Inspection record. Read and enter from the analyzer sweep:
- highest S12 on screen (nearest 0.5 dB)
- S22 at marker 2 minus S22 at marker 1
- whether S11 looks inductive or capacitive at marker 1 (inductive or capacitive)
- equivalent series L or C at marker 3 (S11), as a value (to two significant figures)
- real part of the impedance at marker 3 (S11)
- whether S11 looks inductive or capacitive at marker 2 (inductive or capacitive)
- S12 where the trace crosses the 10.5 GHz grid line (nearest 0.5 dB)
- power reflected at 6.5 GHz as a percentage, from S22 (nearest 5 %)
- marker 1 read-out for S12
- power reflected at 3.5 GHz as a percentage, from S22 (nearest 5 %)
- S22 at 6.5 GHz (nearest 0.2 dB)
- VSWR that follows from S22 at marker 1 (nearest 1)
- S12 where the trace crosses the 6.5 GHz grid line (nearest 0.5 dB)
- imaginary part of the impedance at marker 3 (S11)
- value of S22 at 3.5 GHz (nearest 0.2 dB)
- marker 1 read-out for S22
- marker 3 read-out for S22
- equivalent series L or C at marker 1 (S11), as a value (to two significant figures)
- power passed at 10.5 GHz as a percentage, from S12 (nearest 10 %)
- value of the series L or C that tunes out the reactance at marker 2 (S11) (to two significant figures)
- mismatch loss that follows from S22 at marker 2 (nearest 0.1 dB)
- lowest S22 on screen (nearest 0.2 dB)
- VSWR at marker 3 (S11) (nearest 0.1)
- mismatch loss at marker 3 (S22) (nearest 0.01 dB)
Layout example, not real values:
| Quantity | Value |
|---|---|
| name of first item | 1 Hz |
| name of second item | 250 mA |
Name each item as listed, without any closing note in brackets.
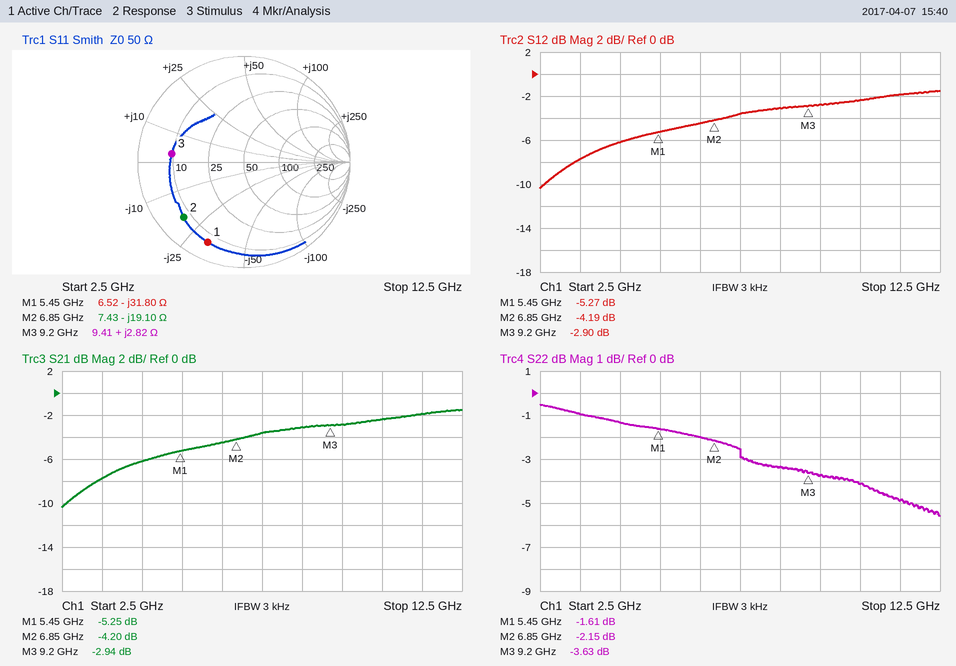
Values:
| Quantity | Value |
|---|---|
| highest S12 on screen | -1.5 dB |
| S22 at marker 2 minus S22 at marker 1 | -0.54 dB |
| whether S11 looks inductive or capacitive at marker 1 | capacitive |
| equivalent series L or C at marker 3 (S11), as a value | 49 pH |
| real part of the impedance at marker 3 | 9.41 Ω |
| whether S11 looks inductive or capacitive at marker 2 | capacitive |
| S12 where the trace crosses the 10.5 GHz grid line | -2.5 dB |
| power reflected at 6.5 GHz as a percentage, from S22 | 65 % |
| marker 1 read-out for S12 | -5.27 dB |
| power reflected at 3.5 GHz as a percentage, from S22 | 80 % |
| S22 at 6.5 GHz | -2.0 dB |
| VSWR that follows from S22 at marker 1 | 11 |
| S12 where the trace crosses the 6.5 GHz grid line | -4.5 dB |
| imaginary part of the impedance at marker 3 | +2.82 Ω |
| value of S22 at 3.5 GHz | -1.0 dB |
| marker 1 read-out for S22 | -1.61 dB |
| marker 3 read-out for S22 | -3.63 dB |
| equivalent series L or C at marker 1 (S11), as a value | 920 fF |
| power passed at 10.5 GHz as a percentage, from S12 | 60 % |
| value of the series L or C that tunes out the reactance at marker 2 (S11) | 440 pH |
| mismatch loss that follows from S22 at marker 2 | 4.1 dB |
| lowest S22 on screen | -5.6 dB |
| VSWR at marker 3 (S11) | 5.3 |
| mismatch loss at marker 3 (S22) | 2.47 dB |
